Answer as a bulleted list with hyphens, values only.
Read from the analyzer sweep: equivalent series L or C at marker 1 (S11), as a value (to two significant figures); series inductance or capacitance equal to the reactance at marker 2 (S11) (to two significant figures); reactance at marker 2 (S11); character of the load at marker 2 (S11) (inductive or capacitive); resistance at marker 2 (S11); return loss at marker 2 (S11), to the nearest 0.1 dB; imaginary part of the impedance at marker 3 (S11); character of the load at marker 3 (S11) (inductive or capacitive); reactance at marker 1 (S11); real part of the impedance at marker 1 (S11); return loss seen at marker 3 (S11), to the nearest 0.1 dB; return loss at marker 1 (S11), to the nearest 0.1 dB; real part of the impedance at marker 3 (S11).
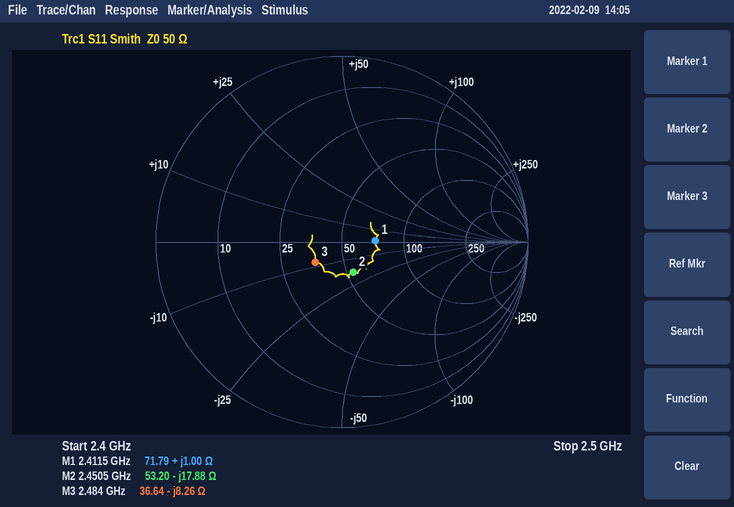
- 66 pH
- 3.6 pF
- -17.88 Ω
- capacitive
- 53.20 Ω
- 15.2 dB
- -8.26 Ω
- capacitive
- +1.00 Ω
- 71.79 Ω
- 14.9 dB
- 14.9 dB
- 36.64 Ω
